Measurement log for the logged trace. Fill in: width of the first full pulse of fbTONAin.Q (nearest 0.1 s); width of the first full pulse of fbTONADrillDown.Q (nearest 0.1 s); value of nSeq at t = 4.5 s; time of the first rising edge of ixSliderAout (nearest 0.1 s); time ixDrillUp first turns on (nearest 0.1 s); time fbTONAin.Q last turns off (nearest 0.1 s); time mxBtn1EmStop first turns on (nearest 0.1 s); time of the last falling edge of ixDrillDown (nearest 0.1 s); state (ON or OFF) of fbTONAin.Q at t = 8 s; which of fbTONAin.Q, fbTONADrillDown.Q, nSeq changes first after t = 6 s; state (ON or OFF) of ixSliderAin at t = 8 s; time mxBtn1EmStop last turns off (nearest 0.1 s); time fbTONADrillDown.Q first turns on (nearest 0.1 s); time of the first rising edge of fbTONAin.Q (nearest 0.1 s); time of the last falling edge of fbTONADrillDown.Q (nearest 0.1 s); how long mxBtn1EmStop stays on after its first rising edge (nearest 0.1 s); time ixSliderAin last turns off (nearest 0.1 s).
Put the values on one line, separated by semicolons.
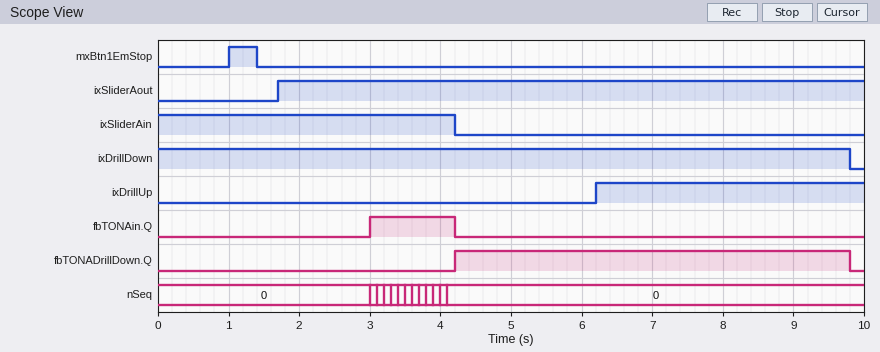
1.2 s; 5.6 s; 0; 1.7 s; 6.2 s; 4.2 s; 1.0 s; 9.8 s; OFF; fbTONADrillDown.Q; OFF; 1.4 s; 4.2 s; 3.0 s; 9.8 s; 0.4 s; 4.2 s
